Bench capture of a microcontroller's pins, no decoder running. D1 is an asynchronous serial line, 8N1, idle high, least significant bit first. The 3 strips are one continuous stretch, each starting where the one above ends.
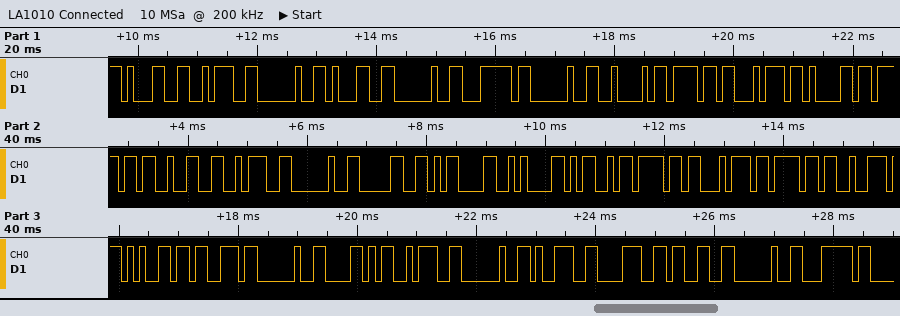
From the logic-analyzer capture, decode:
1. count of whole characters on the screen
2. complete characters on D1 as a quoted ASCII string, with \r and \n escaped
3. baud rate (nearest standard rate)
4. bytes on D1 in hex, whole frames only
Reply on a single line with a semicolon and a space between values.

34; "1: 1 | Botao2: 0\r\nMotores X: 983 |"; 9600 baud; 31 3A 20 31 20 7C 20 42 6F 74 61 6F 32 3A 20 30 0D 0A 4D 6F 74 6F 72 65 73 20 58 3A 20 39 38 33 20 7C
